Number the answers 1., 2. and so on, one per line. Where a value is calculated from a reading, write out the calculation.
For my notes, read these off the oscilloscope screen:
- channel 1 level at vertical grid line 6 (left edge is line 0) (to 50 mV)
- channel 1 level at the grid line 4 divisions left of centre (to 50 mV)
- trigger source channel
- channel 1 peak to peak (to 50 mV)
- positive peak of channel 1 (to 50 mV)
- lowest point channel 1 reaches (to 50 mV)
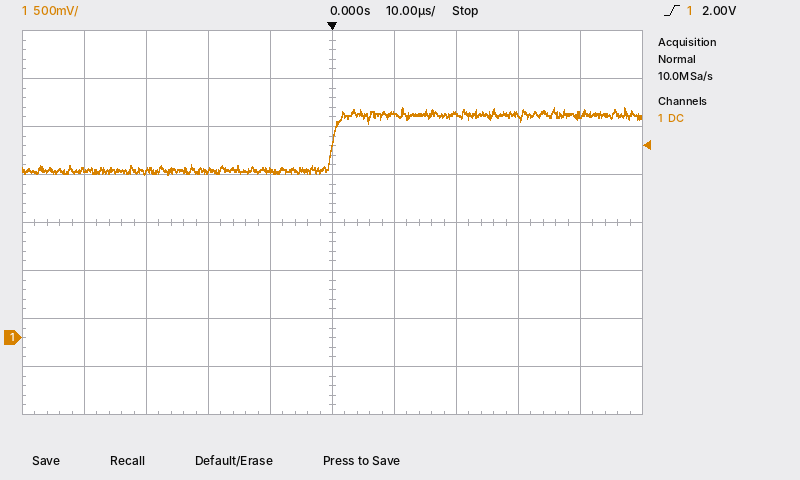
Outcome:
1. 2.35 V
2. 1.75 V
3. channel 1
4. 2.40 V − (1.70 V) = 700 mV
5. 2.40 V
6. 1.70 V
